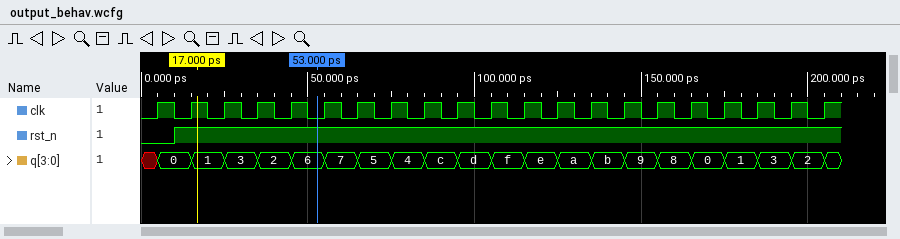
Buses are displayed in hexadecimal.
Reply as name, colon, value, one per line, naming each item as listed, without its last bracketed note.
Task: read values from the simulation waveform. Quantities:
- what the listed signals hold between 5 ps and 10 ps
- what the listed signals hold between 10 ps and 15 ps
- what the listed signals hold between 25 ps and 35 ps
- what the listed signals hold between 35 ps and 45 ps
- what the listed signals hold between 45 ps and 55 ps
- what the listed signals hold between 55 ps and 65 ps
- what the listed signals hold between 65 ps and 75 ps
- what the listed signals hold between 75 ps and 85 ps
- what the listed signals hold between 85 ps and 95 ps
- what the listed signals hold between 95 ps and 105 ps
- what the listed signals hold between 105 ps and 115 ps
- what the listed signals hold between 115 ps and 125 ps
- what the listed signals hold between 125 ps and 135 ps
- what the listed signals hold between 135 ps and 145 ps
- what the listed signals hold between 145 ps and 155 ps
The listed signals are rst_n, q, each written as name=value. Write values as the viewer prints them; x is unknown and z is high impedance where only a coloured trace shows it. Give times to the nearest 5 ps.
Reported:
what the listed signals hold between 5 ps and 10 ps: rst_n=0, q=0
what the listed signals hold between 10 ps and 15 ps: rst_n=1, q=0
what the listed signals hold between 25 ps and 35 ps: rst_n=1, q=3
what the listed signals hold between 35 ps and 45 ps: rst_n=1, q=2
what the listed signals hold between 45 ps and 55 ps: rst_n=1, q=6
what the listed signals hold between 55 ps and 65 ps: rst_n=1, q=7
what the listed signals hold between 65 ps and 75 ps: rst_n=1, q=5
what the listed signals hold between 75 ps and 85 ps: rst_n=1, q=4
what the listed signals hold between 85 ps and 95 ps: rst_n=1, q=c
what the listed signals hold between 95 ps and 105 ps: rst_n=1, q=d
what the listed signals hold between 105 ps and 115 ps: rst_n=1, q=f
what the listed signals hold between 115 ps and 125 ps: rst_n=1, q=e
what the listed signals hold between 125 ps and 135 ps: rst_n=1, q=a
what the listed signals hold between 135 ps and 145 ps: rst_n=1, q=b
what the listed signals hold between 145 ps and 155 ps: rst_n=1, q=9
